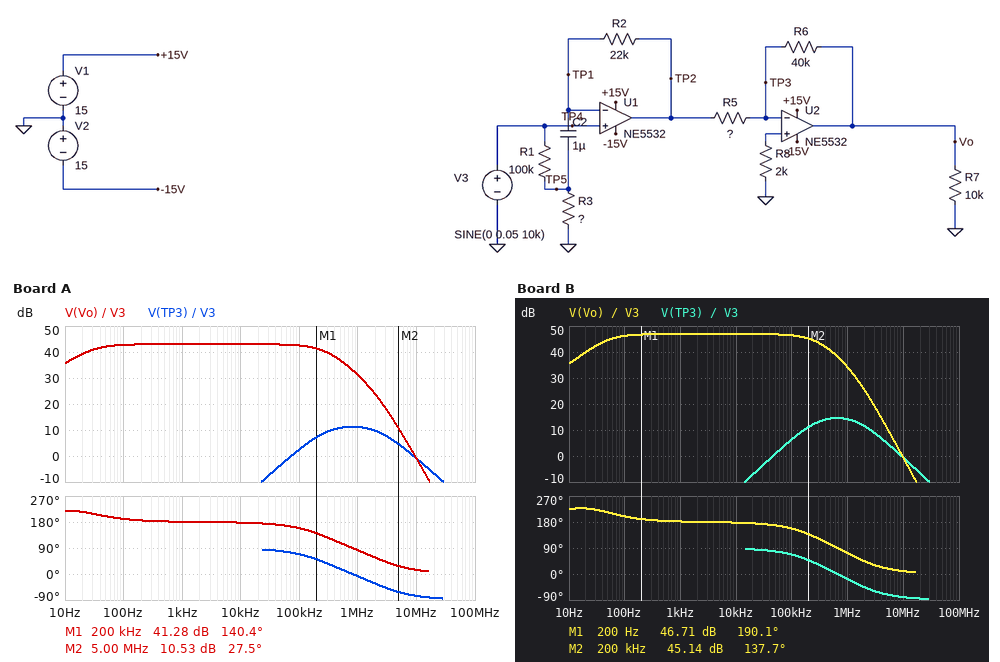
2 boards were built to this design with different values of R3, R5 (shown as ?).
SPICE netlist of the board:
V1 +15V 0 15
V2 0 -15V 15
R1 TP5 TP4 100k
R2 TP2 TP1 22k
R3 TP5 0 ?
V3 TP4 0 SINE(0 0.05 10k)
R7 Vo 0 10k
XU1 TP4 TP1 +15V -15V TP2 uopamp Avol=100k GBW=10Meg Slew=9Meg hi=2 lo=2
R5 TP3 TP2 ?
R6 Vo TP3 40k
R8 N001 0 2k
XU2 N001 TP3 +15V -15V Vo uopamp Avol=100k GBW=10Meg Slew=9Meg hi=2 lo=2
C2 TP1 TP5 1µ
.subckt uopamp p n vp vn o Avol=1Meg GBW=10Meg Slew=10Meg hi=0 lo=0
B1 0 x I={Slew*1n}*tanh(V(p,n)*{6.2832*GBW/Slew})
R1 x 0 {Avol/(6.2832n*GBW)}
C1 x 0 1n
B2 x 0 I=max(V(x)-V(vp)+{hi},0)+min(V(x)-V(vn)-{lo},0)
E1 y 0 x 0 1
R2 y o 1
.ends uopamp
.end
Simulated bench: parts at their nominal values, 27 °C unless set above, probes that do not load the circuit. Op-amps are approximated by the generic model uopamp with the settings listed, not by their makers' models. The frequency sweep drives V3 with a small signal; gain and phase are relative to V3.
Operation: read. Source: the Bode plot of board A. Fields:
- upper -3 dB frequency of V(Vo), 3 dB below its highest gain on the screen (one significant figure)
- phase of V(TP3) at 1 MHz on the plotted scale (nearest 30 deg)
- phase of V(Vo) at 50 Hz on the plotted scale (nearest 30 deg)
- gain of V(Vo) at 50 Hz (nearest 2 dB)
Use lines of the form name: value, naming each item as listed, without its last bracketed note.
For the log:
upper -3 dB frequency of V(Vo), 3 dB below its highest gain on the screen: 300 kHz
phase of V(TP3) at 1 MHz on the plotted scale: 0 deg
phase of V(Vo) at 50 Hz on the plotted scale: 210 deg
gain of V(Vo) at 50 Hz: 42 dB
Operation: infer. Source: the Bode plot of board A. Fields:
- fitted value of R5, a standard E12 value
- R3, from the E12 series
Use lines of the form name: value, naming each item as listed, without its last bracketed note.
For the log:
fitted value of R5, a standard E12 value: 1.2 kΩ
R3, from the E12 series: 6.8 kΩ
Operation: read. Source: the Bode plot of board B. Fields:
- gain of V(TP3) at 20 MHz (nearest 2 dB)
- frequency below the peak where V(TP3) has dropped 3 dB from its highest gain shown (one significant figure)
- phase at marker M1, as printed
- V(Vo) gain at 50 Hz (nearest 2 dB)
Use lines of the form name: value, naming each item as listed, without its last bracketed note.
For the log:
gain of V(TP3) at 20 MHz: -6 dB
frequency below the peak where V(TP3) has dropped 3 dB from its highest gain shown: 200 kHz
phase at marker M1, as printed: 190.1 deg
V(Vo) gain at 50 Hz: 44 dB
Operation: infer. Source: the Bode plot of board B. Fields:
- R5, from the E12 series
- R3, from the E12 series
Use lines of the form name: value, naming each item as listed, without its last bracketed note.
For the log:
R5, from the E12 series: 1.2 kΩ
R3, from the E12 series: 3.9 kΩ
